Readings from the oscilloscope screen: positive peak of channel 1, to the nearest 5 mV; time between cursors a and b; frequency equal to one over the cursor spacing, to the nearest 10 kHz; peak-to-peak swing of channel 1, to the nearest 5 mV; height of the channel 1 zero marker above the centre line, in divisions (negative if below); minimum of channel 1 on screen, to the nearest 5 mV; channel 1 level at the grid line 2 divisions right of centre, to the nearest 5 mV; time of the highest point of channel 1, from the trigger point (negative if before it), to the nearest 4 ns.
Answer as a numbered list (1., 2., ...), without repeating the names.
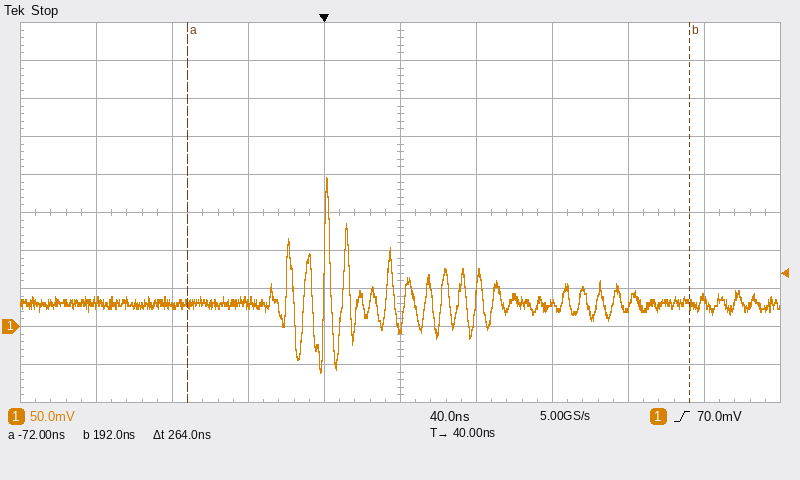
1. 195 mV
2. 264 ns
3. 3.79 MHz
4. 255 mV
5. -3.0 div
6. -60 mV
7. 30 mV
8. 0 ns
